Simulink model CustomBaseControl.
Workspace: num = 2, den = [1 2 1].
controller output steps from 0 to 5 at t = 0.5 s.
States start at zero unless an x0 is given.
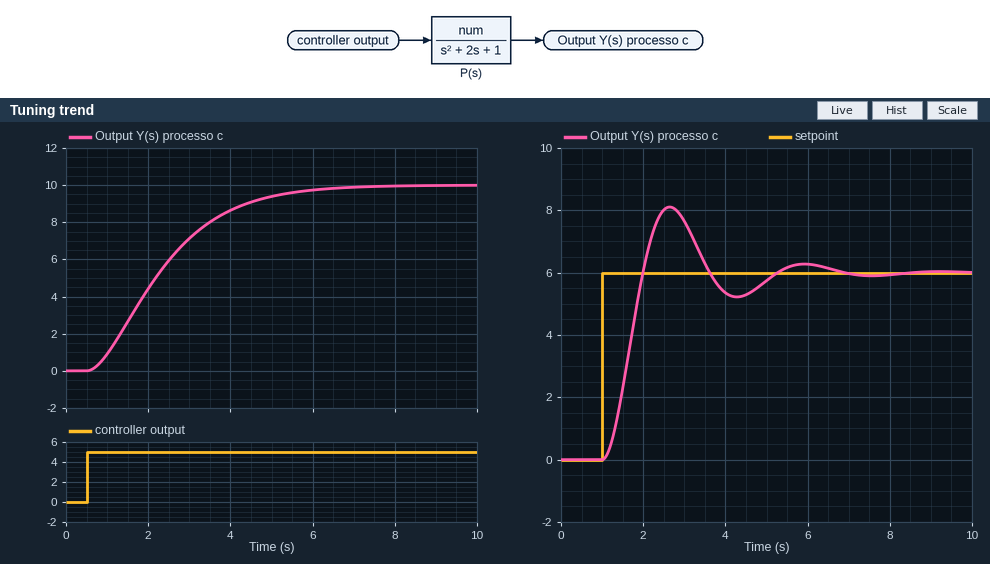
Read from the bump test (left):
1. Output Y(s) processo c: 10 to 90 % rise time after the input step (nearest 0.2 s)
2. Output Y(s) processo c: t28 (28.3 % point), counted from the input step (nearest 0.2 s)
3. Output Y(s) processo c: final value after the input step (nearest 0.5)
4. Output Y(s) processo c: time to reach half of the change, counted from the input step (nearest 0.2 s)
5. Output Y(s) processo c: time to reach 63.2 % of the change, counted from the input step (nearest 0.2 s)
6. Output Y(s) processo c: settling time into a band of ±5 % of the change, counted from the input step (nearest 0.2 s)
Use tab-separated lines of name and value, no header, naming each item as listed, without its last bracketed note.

Output Y(s) processo c: 10 to 90 % rise time after the input step	3.4 s
Output Y(s) processo c: t28 (28.3 % point), counted from the input step	1.0 s
Output Y(s) processo c: final value after the input step	10.0
Output Y(s) processo c: time to reach half of the change, counted from the input step	1.6 s
Output Y(s) processo c: time to reach 63.2 % of the change, counted from the input step	2.2 s
Output Y(s) processo c: settling time into a band of ±5 % of the change, counted from the input step	4.8 s
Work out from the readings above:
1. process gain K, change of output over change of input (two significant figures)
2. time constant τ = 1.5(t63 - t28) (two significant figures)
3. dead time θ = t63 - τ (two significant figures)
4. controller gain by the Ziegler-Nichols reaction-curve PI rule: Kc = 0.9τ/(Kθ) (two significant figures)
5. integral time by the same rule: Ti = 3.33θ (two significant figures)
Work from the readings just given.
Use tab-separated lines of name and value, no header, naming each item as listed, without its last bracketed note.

process gain K, change of output over change of input	2.0
time constant τ = 1.5(t63 - t28)	1.8 s
dead time θ = t63 - τ	0.40 s
controller gain by the Ziegler-Nichols reaction-curve PI rule: Kc = 0.9τ/(Kθ)	2.0
integral time by the same rule: Ti = 3.33θ	1.3 s
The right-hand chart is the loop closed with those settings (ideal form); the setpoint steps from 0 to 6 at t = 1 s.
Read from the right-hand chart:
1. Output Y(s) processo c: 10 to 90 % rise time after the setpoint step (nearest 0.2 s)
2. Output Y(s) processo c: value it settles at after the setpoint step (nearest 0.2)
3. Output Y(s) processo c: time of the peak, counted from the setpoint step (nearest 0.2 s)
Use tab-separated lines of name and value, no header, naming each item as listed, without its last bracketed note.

Output Y(s) processo c: 10 to 90 % rise time after the setpoint step	0.6 s
Output Y(s) processo c: value it settles at after the setpoint step	6.0
Output Y(s) processo c: time of the peak, counted from the setpoint step	1.6 s
